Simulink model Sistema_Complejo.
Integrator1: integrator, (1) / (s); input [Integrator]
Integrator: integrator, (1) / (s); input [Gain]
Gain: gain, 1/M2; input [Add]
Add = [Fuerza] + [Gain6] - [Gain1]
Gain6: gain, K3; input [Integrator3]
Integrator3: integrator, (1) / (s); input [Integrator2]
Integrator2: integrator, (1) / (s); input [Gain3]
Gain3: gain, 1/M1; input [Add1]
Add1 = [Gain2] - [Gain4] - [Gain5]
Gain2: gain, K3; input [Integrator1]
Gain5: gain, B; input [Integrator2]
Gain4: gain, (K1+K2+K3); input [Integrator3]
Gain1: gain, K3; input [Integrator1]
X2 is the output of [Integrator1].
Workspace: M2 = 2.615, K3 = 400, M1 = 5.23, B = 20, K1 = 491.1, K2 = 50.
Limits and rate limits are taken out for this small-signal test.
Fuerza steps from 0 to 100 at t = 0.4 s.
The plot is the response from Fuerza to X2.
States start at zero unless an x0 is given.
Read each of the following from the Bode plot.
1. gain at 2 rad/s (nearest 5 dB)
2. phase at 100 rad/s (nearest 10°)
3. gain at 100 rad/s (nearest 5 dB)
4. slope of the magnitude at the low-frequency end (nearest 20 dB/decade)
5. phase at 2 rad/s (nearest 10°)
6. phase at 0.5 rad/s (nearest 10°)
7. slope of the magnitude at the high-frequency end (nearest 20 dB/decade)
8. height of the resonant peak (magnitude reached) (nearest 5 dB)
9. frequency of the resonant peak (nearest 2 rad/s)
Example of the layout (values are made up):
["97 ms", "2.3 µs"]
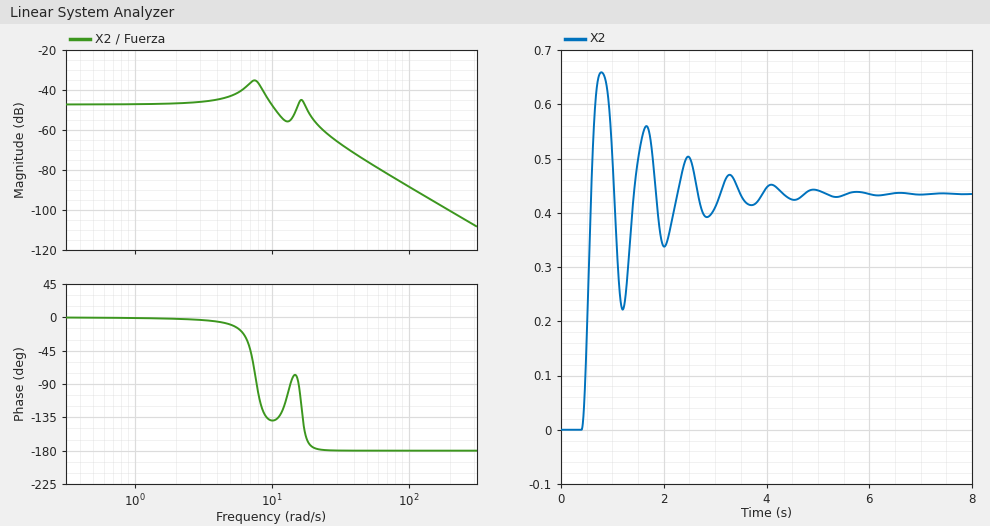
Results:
["-45 dB", "-180°", "-90 dB", "0 dB/decade", "0°", "0°", "-40 dB/decade", "-35 dB", "8 rad/s"]
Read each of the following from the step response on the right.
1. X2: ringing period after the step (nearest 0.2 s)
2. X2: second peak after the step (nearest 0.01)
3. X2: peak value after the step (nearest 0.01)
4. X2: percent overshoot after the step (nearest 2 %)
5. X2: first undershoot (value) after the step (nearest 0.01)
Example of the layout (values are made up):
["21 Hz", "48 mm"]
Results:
["0.8 s", "0.56", "0.66", "52 %", "0.22"]
